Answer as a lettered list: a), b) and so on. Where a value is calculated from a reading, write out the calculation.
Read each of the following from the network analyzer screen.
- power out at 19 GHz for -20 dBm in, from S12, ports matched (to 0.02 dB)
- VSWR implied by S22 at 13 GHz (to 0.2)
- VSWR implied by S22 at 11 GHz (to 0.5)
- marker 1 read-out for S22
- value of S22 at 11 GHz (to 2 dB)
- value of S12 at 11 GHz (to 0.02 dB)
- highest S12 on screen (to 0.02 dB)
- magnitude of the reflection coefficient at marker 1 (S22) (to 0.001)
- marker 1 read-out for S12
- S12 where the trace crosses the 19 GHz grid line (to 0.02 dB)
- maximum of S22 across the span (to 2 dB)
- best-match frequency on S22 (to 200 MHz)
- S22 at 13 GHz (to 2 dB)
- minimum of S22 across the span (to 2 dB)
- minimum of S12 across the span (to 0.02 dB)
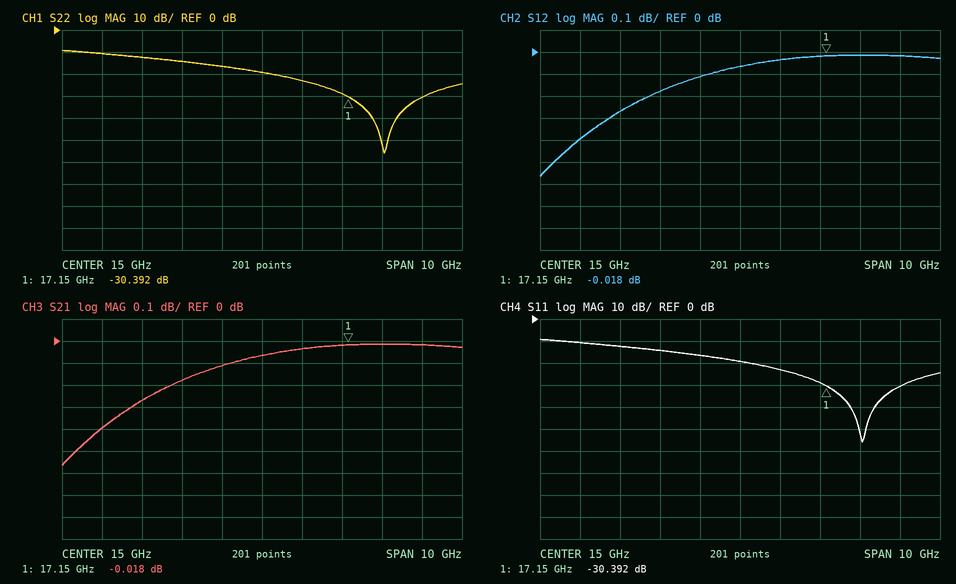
a) -20 dBm + (-0.02 dB) = -20.02 dBm
b) |Γ| = 10^(-14/20) = 0.1995; VSWR = (1 + 0.1995)/(1 − 0.1995) ≈ 1.50, so 1.4 to the nearest 0.2
c) |Γ| = 10^(-10/20) = 0.3162; VSWR = (1 + 0.3162)/(1 − 0.3162) ≈ 1.92, so 2.0 to the nearest 0.5
d) -30.392 dB
e) -10 dB
f) -0.40 dB
g) -0.02 dB
h) 10^(-30.392/20) ≈ 0.030
i) -0.018 dB
j) -0.02 dB
k) -10 dB
l) 18.0 GHz
m) -14 dB
n) -56 dB
o) -0.56 dB
